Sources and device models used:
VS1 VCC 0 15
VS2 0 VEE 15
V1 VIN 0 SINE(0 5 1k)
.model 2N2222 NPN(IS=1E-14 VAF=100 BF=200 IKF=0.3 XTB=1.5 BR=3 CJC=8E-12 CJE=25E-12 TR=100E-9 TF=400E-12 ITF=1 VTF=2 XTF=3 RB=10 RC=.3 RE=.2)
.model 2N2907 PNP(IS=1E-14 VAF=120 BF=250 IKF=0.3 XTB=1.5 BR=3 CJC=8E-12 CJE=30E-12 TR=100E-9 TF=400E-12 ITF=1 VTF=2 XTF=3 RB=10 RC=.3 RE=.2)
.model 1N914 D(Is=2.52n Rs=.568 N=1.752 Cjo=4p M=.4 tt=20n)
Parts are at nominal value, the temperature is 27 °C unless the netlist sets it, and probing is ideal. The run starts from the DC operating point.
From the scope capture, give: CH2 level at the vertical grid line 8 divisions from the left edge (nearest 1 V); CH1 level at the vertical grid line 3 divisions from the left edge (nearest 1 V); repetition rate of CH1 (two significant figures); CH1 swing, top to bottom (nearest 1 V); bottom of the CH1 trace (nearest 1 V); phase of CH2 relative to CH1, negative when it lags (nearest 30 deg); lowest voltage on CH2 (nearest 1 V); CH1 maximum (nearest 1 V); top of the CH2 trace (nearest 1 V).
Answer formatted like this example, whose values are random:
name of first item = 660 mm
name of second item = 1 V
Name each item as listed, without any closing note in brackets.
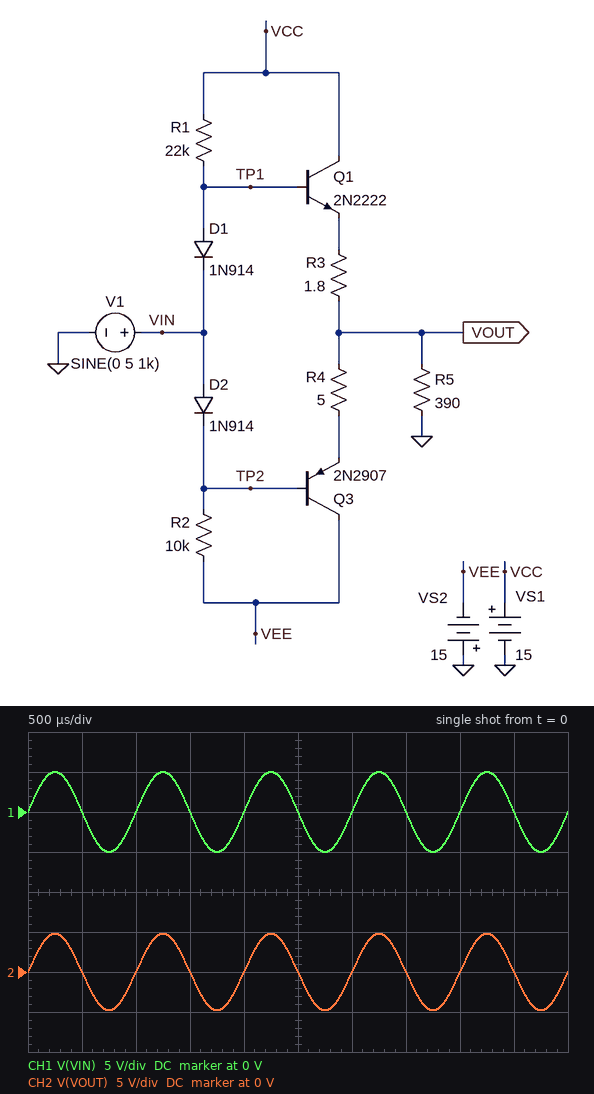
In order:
CH2 level at the vertical grid line 8 divisions from the left edge = 0 V
CH1 level at the vertical grid line 3 divisions from the left edge = 0 V
repetition rate of CH1 = 1.0 kHz
CH1 swing, top to bottom = 10 V
bottom of the CH1 trace = -5 V
phase of CH2 relative to CH1, negative when it lags = 0 deg
lowest voltage on CH2 = -5 V
CH1 maximum = 5 V
top of the CH2 trace = 5 V
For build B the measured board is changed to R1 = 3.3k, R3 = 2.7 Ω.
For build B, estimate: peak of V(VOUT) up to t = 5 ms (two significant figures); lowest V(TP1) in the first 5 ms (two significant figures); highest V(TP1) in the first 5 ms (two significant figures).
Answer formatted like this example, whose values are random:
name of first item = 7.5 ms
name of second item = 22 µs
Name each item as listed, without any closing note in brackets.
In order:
peak of V(VOUT) up to t = 5 ms = 4.9 V
lowest V(TP1) in the first 5 ms = -4.3 V
highest V(TP1) in the first 5 ms = 5.6 V
